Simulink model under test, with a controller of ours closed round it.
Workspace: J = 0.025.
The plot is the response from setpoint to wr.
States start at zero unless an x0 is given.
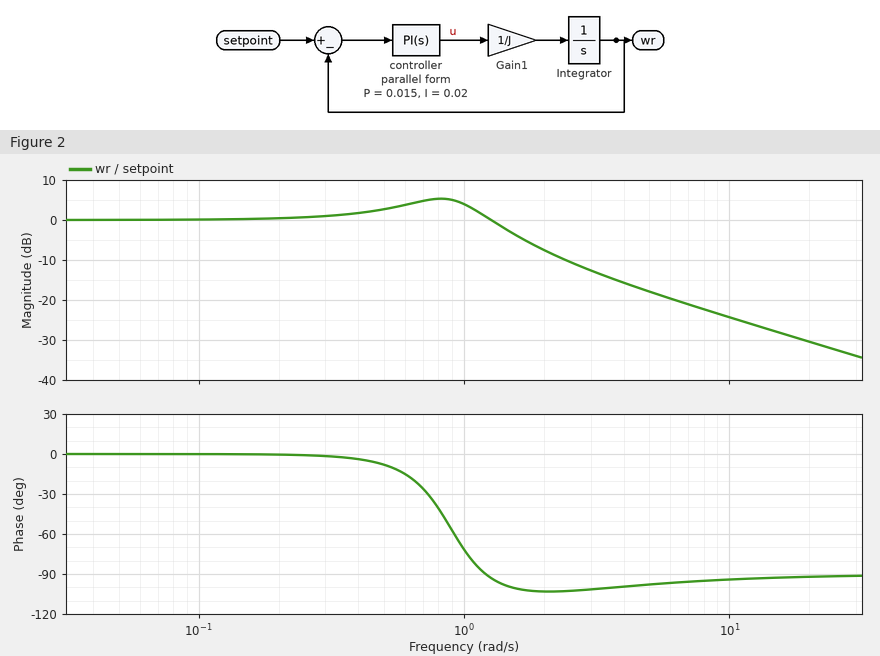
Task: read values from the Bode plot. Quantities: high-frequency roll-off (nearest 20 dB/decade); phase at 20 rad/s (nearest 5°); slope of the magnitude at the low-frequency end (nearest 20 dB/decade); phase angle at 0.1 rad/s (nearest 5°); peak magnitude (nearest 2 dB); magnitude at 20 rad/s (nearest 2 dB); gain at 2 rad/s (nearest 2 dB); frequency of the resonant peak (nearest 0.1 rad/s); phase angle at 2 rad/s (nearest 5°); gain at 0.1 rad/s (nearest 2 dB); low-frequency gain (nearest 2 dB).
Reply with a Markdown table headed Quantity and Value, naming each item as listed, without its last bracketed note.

| Quantity | Value |
|---|---|
| high-frequency roll-off | -20 dB/decade |
| phase at 20 rad/s | -90° |
| slope of the magnitude at the low-frequency end | 0 dB/decade |
| phase angle at 0.1 rad/s | 0° |
| peak magnitude | 6 dB |
| magnitude at 20 rad/s | -30 dB |
| gain at 2 rad/s | -8 dB |
| frequency of the resonant peak | 0.8 rad/s |
| phase angle at 2 rad/s | -105° |
| gain at 0.1 rad/s | 0 dB |
| low-frequency gain | 0 dB |
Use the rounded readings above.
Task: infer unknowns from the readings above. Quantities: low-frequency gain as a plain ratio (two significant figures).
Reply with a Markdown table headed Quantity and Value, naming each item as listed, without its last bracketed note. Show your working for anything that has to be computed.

| Quantity | Value |
|---|---|
| low-frequency gain as a plain ratio | 10^(0 / 20) = 1.0 |
